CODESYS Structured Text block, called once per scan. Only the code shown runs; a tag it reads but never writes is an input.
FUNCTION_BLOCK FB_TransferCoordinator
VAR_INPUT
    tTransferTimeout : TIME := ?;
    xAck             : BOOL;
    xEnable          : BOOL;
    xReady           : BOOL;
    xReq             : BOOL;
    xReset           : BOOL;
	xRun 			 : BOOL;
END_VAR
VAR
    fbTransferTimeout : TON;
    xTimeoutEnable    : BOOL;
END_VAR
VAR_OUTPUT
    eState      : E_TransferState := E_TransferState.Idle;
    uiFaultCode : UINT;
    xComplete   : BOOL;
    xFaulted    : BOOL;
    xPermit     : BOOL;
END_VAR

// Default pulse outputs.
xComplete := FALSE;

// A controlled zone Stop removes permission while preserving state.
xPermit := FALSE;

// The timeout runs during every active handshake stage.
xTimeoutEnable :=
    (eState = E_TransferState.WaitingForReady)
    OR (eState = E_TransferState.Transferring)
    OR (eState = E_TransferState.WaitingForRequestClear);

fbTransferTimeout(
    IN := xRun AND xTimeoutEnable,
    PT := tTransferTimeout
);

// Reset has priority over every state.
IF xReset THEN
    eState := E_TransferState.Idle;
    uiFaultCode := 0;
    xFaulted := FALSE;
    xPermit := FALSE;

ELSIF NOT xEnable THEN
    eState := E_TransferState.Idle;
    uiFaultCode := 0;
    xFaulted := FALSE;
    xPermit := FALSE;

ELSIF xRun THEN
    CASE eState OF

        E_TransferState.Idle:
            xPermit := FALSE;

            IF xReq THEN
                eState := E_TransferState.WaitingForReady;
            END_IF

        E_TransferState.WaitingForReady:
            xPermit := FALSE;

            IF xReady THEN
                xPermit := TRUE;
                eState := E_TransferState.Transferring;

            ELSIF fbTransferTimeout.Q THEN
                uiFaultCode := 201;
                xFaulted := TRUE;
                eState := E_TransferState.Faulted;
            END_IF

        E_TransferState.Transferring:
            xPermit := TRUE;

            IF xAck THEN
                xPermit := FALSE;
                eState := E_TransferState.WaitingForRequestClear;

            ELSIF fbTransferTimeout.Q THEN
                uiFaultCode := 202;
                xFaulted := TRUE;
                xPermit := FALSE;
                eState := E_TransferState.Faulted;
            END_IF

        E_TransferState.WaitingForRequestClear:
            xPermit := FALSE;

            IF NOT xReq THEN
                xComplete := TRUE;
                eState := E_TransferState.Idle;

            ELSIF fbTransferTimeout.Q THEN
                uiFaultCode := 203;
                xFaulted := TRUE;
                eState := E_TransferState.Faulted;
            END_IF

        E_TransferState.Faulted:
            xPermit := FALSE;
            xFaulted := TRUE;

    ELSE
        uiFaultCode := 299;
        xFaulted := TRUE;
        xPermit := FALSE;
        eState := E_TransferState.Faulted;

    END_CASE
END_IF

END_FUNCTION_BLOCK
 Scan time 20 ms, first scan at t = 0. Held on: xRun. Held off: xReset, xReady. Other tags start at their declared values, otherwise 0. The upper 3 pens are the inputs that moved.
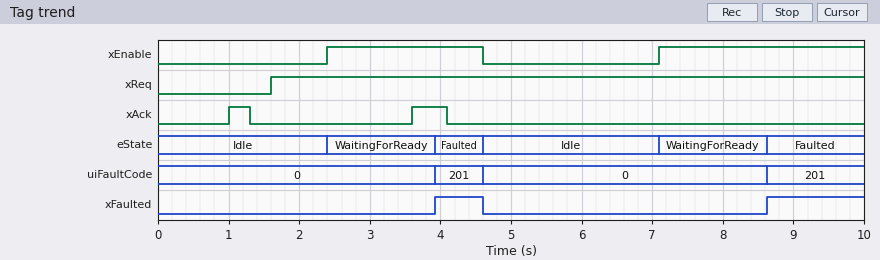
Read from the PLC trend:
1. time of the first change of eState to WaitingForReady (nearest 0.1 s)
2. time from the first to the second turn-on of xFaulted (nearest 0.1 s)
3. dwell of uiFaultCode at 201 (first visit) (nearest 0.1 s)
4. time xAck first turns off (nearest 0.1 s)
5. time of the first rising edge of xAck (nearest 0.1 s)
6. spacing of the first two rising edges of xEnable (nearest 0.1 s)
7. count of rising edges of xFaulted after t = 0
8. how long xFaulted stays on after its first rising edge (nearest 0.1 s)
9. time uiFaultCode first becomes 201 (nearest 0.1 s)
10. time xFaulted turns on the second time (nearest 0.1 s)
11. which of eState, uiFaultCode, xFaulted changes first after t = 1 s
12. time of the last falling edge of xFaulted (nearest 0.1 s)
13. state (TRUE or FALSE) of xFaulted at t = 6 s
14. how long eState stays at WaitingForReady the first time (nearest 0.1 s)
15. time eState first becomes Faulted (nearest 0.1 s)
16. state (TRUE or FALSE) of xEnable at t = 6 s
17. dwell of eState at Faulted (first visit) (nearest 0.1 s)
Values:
2.4 s
4.7 s
0.7 s
1.3 s
1.0 s
4.7 s
2
0.7 s
3.9 s
8.6 s
eState
4.6 s
FALSE
1.5 s
3.9 s
FALSE
0.7 s
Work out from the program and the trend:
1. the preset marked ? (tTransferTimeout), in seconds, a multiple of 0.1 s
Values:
1.5 s
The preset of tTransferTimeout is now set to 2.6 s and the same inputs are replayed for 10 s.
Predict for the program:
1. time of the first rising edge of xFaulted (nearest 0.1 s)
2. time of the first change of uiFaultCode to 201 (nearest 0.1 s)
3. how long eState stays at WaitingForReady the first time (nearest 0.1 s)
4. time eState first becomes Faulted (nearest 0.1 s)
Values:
9.7 s
9.7 s
2.2 s
9.7 s
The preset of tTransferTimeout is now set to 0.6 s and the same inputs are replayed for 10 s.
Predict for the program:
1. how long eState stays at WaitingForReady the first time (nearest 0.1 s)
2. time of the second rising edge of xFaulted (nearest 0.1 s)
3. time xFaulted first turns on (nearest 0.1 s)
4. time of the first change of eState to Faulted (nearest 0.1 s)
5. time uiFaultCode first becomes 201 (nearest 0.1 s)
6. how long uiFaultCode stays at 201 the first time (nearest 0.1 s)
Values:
0.6 s
7.7 s
3.0 s
3.0 s
3.0 s
1.6 s
